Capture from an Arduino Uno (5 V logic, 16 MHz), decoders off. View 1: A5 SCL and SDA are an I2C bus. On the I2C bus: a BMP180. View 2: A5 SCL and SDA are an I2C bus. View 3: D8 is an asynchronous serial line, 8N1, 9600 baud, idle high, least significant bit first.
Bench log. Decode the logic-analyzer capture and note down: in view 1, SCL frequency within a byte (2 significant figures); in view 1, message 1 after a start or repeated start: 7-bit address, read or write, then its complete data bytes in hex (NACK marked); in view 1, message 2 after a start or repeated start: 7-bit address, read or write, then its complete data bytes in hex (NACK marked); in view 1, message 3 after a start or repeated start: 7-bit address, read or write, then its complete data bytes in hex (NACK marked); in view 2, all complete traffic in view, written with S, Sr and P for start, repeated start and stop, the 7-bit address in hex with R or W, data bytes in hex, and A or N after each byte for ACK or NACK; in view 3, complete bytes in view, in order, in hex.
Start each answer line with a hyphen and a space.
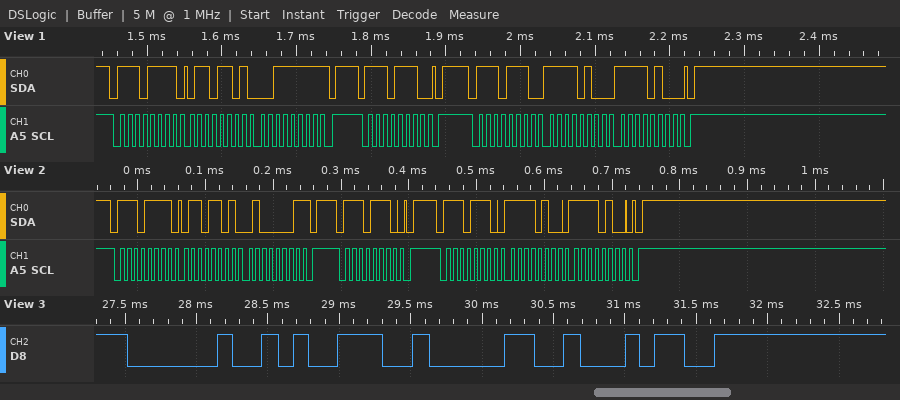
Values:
- 100 kHz
- 0x77 read: 6D 3F NACK
- 0x77 write
- 0x77 write: F4 F4
- S 77R A 6D A 41 N P S 77W A P S 77W A F4 A F4 A P
- 20 39 30 34
